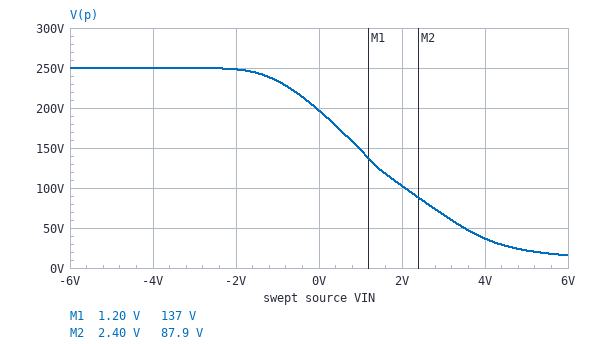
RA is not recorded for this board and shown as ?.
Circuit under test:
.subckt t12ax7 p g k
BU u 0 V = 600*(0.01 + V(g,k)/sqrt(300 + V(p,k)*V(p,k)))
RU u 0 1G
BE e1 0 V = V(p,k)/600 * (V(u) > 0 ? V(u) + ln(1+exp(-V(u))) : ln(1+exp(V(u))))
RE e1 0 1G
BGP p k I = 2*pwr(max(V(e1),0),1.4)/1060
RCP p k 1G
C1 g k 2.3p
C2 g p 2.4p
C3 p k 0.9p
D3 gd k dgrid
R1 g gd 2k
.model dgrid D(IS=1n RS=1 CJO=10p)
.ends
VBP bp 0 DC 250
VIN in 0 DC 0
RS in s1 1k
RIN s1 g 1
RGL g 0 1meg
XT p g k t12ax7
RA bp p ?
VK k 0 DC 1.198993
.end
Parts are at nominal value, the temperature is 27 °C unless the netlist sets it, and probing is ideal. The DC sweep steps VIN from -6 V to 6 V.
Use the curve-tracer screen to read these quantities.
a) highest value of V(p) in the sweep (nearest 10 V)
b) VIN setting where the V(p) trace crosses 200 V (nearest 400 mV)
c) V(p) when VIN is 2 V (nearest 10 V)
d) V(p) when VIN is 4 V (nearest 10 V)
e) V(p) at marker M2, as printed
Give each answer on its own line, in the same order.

250 V
0 V
100 V
40 V
87.9 V
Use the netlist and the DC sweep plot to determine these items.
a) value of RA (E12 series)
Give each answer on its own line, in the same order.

39 kΩ
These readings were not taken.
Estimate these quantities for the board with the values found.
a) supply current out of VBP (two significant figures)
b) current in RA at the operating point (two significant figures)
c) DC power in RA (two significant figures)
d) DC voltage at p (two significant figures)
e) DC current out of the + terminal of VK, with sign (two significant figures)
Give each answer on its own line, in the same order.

1.4 mA
1.4 mA
72 mW
200 V
-1.4 mA
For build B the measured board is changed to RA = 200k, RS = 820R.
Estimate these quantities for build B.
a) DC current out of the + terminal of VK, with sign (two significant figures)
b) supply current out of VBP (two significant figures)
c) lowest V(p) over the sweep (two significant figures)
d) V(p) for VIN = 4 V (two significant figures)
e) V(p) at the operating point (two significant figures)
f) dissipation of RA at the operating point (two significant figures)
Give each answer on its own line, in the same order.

-490 µA
490 µA
4.7 V
7.1 V
150 V
48 mW
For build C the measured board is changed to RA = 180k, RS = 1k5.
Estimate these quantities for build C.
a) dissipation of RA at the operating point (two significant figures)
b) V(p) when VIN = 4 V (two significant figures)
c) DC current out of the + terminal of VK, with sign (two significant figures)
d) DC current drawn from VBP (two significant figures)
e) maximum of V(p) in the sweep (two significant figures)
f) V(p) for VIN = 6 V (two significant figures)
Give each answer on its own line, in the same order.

50 mW
8.9 V
-530 µA
530 µA
250 V
5.8 V
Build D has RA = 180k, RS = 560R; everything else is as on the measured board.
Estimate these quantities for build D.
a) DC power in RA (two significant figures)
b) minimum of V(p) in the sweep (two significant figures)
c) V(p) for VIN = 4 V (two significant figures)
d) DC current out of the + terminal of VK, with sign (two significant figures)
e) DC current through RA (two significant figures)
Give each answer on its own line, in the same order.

50 mW
4.7 V
7.1 V
-530 µA
530 µA
